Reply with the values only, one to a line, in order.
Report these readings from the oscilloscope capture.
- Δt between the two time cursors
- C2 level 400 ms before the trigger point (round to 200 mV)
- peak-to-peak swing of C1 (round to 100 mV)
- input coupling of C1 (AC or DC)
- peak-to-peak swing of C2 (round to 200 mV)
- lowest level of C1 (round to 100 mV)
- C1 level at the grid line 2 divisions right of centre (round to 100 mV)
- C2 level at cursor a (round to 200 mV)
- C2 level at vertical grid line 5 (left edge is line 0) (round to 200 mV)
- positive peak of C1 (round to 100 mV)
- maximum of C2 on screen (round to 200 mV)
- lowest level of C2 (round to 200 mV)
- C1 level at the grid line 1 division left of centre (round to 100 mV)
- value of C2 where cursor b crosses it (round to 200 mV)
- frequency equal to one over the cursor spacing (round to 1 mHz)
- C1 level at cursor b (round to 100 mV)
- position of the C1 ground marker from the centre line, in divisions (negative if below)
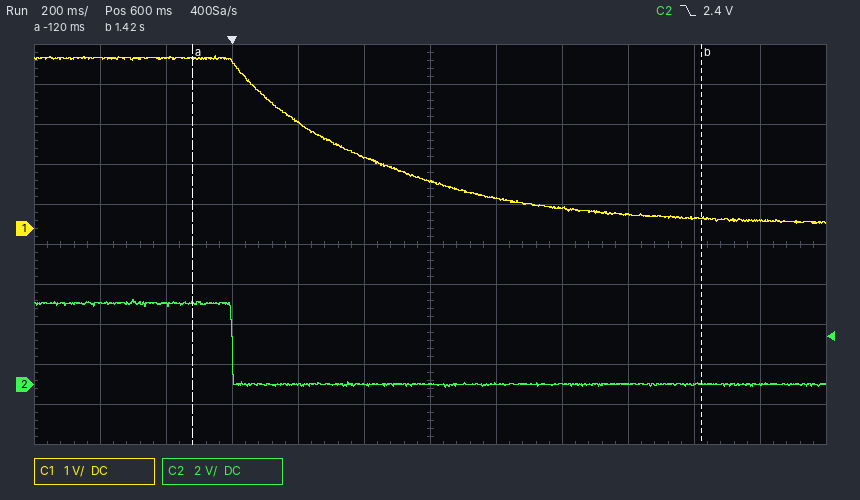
1.54 s
4.0 V
4.2 V
DC
4.4 V
100 mV
500 mV
4.0 V
0.0 V
4.3 V
4.2 V
-200 mV
1.8 V
0.0 V
649 mHz
300 mV
+0.4 div
